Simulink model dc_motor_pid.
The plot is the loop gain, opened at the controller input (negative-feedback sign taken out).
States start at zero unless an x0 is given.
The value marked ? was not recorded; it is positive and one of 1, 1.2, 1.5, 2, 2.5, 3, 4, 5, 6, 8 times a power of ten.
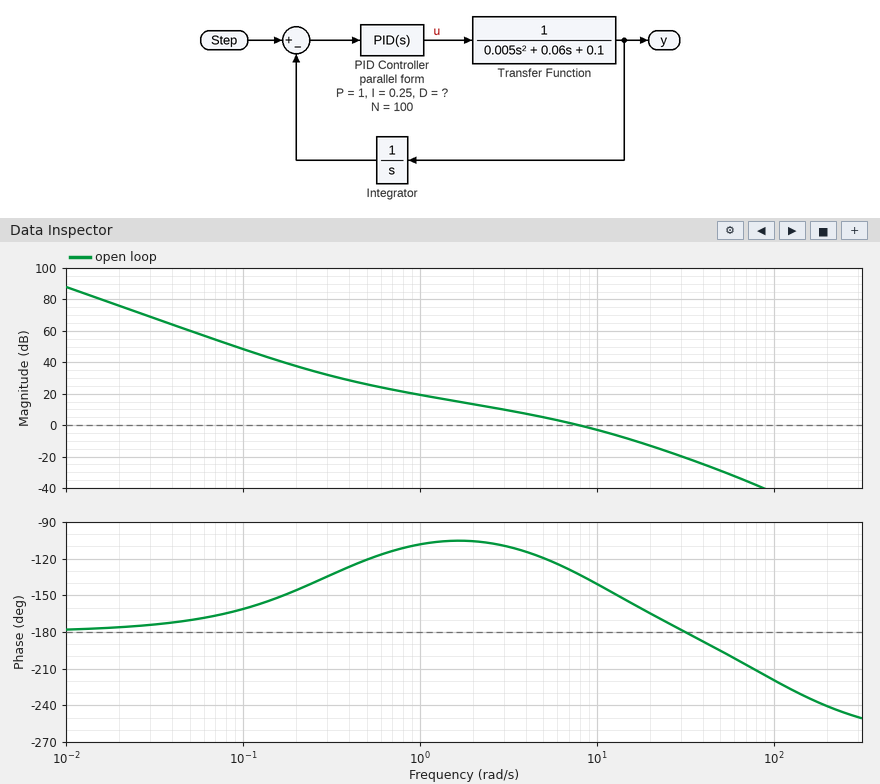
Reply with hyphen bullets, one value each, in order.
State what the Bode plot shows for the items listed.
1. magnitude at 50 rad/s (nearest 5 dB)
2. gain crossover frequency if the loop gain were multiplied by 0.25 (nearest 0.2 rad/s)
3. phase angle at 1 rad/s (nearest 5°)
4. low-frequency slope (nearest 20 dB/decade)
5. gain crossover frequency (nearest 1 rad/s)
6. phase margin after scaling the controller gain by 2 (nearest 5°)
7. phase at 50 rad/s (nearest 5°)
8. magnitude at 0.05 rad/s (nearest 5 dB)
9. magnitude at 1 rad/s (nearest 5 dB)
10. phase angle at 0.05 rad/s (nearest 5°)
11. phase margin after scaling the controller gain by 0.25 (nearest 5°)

- -30 dB
- 2.4 rad/s
- -110°
- -40 dB/decade
- 8 rad/s
- 30°
- -195°
- 60 dB
- 20 dB
- -170°
- 75°
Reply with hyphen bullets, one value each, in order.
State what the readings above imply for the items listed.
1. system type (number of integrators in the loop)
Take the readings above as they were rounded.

- 2
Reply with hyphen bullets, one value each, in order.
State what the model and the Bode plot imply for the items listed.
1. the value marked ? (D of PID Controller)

- 0.5
